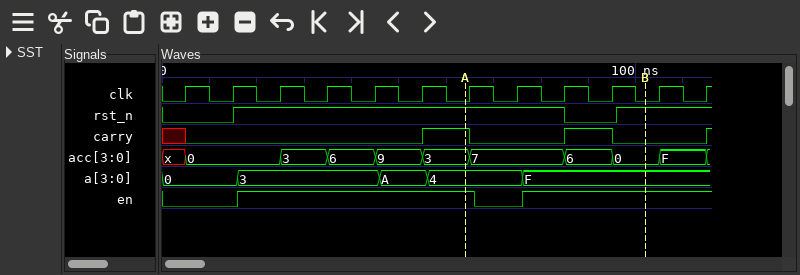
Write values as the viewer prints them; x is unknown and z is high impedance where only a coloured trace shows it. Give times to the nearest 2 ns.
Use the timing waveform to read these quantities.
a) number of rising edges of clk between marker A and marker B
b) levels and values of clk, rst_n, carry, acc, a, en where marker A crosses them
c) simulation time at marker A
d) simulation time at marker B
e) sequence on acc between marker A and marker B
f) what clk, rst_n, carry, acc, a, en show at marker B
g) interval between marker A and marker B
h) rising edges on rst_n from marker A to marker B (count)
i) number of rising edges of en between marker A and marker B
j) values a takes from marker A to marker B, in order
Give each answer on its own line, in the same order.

4
clk=0, rst_n=1, carry=1, acc=3, a=4, en=1
64 ns
102 ns
3, 7, 6, 0
clk=0, rst_n=1, carry=0, acc=0, a=F, en=1
38 ns
1
1
4, F
